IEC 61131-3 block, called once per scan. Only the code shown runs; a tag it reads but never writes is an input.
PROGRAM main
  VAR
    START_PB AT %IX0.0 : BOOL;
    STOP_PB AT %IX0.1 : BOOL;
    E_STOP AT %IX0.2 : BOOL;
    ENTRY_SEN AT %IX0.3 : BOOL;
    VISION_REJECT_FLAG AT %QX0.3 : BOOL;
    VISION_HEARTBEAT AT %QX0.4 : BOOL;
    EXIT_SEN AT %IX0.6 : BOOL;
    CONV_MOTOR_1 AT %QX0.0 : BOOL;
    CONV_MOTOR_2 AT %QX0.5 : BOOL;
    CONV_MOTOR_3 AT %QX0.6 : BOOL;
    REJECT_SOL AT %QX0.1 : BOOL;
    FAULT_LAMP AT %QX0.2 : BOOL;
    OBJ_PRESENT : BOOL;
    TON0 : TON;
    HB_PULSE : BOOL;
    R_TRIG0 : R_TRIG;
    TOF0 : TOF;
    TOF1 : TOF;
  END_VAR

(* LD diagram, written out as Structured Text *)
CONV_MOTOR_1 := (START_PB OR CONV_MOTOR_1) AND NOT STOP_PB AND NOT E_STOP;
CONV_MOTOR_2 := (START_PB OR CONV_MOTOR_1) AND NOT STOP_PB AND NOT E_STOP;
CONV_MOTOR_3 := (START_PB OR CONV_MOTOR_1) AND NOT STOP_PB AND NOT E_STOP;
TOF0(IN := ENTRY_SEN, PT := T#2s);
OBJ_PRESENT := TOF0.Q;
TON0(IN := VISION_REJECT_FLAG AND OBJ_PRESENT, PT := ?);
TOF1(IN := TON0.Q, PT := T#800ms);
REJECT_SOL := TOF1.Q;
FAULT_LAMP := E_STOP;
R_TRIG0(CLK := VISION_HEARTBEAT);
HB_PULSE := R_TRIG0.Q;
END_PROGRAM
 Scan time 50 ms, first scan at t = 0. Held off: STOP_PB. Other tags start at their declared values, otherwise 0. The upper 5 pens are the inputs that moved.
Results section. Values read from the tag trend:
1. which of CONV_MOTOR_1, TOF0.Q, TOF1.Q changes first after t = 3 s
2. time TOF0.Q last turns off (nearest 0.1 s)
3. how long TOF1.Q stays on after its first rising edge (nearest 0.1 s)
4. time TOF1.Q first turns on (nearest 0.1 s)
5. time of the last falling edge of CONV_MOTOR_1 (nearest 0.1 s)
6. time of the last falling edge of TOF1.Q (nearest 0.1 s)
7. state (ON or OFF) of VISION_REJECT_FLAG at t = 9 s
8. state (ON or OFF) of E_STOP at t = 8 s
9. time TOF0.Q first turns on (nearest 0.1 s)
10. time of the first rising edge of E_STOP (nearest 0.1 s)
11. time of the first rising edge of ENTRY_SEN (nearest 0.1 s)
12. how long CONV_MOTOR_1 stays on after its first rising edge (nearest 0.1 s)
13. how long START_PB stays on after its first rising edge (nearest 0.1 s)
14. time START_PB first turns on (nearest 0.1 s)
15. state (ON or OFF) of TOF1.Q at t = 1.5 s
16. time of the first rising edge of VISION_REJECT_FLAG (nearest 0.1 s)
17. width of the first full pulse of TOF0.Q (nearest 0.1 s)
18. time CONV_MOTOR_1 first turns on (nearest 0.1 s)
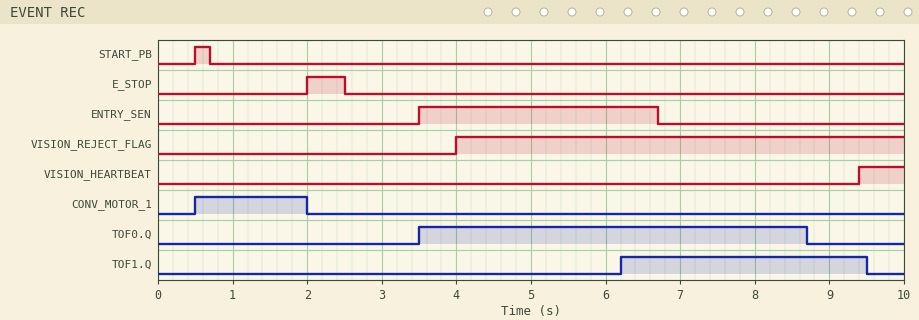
TOF0.Q
8.7 s
3.3 s
6.2 s
2.0 s
9.5 s
ON
OFF
3.5 s
2.0 s
3.5 s
1.5 s
0.2 s
0.5 s
OFF
4.0 s
5.2 s
0.5 s
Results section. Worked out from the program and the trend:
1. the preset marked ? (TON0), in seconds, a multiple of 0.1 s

2.2 s
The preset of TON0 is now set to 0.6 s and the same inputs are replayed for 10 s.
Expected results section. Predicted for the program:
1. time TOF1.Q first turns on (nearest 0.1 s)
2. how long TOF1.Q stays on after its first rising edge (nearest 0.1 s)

4.6 s
4.9 s
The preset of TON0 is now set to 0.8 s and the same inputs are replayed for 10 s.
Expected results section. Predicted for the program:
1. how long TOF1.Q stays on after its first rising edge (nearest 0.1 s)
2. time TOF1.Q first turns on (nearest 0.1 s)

4.7 s
4.8 s
